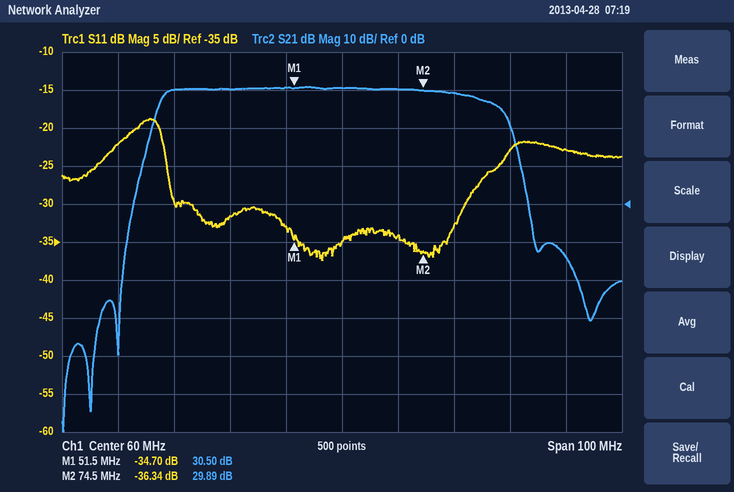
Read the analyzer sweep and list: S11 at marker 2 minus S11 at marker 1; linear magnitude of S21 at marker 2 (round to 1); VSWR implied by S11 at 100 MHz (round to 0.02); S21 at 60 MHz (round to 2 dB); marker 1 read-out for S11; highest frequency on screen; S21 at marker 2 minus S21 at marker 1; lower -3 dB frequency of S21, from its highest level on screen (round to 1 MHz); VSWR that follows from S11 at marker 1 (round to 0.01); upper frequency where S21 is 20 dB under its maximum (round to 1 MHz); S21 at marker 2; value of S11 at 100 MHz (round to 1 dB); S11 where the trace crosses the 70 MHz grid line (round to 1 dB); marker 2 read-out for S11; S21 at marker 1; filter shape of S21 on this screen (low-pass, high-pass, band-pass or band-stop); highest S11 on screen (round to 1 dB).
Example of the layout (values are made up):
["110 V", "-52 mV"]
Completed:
["-1.64 dB", "31", "1.16", "30 dB", "-34.70 dB", "110 MHz", "-0.61 dB", "28 MHz", "1.04", "92 MHz", "29.89 dB", "-23 dB", "-34 dB", "-36.34 dB", "30.50 dB", "band-pass", "-19 dB"]
